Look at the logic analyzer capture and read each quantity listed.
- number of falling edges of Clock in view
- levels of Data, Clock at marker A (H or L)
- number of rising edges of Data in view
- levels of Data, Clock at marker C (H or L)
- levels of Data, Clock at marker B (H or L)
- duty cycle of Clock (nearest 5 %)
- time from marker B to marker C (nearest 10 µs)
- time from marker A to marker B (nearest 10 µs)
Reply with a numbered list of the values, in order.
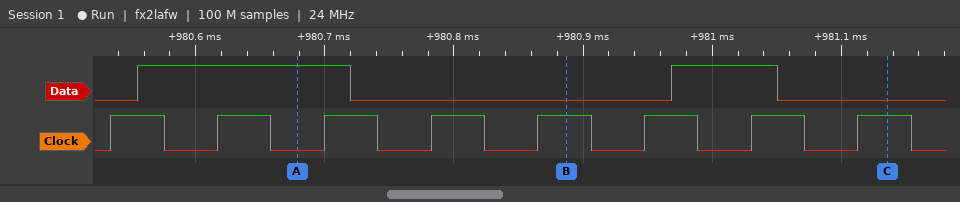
1. 8
2. Data=H, Clock=L
3. 2
4. Data=L, Clock=H
5. Data=L, Clock=H
6. 50 %
7. 250 µs
8. 210 µs
